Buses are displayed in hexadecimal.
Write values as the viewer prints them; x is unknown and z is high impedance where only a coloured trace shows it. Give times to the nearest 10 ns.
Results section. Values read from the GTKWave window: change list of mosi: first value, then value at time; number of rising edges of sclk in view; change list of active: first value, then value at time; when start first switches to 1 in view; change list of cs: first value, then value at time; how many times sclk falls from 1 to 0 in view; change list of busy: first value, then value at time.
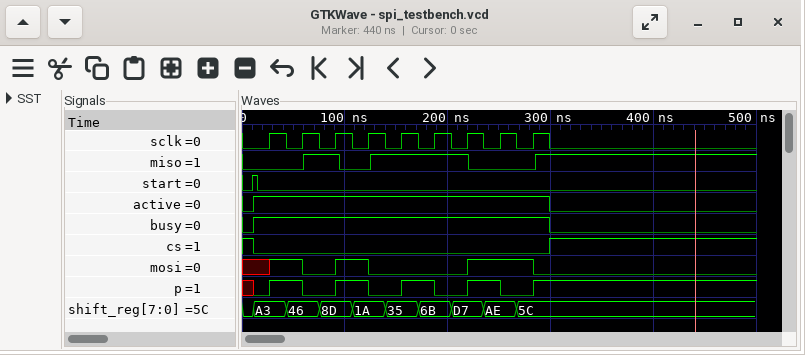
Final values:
x, 1 at 30 ns, 0 at 60 ns, 1 at 90 ns, 0 at 120 ns, 1 at 220 ns, 0 at 280 ns
9
0, 1 at 10 ns, 0 at 300 ns
10 ns
1, 0 at 10 ns, 1 at 300 ns
9
0, 1 at 10 ns, 0 at 300 ns
